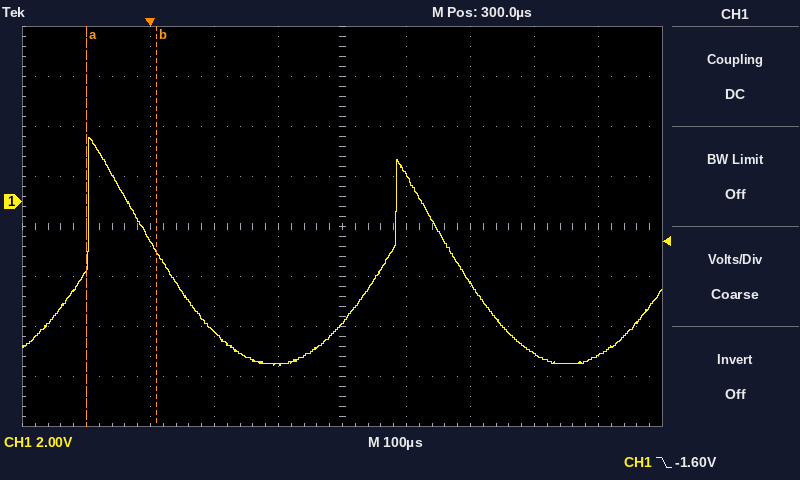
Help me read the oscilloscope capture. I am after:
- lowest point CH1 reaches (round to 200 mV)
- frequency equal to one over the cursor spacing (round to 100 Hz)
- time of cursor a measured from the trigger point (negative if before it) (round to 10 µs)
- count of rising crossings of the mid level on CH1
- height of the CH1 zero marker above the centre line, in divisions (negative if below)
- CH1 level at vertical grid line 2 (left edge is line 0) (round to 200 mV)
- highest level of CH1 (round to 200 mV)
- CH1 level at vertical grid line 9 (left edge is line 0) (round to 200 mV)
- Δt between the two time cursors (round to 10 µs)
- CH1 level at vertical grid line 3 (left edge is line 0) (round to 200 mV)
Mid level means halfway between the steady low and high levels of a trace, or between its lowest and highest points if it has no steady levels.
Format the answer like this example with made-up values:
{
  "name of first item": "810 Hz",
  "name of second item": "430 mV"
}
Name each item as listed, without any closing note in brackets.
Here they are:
{
  "lowest point CH1 reaches": "-6.6 V",
  "frequency equal to one over the cursor spacing": "9.1 kHz",
  "time of cursor a measured from the trigger point (negative if before it)": "-100 µs",
  "count of rising crossings of the mid level on CH1": "2",
  "height of the CH1 zero marker above the centre line, in divisions": "+0.5 div",
  "CH1 level at vertical grid line 2 (left edge is line 0)": "-1.6 V",
  "highest level of CH1": "2.6 V",
  "CH1 level at vertical grid line 9 (left edge is line 0)": "-6.2 V",
  "Δt between the two time cursors": "110 µs",
  "CH1 level at vertical grid line 3 (left edge is line 0)": "-5.2 V"
}
